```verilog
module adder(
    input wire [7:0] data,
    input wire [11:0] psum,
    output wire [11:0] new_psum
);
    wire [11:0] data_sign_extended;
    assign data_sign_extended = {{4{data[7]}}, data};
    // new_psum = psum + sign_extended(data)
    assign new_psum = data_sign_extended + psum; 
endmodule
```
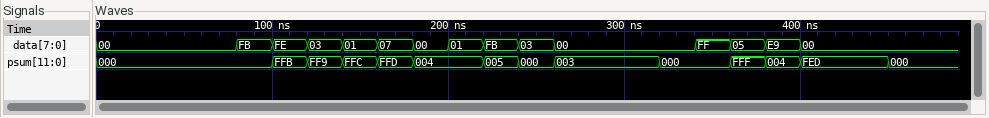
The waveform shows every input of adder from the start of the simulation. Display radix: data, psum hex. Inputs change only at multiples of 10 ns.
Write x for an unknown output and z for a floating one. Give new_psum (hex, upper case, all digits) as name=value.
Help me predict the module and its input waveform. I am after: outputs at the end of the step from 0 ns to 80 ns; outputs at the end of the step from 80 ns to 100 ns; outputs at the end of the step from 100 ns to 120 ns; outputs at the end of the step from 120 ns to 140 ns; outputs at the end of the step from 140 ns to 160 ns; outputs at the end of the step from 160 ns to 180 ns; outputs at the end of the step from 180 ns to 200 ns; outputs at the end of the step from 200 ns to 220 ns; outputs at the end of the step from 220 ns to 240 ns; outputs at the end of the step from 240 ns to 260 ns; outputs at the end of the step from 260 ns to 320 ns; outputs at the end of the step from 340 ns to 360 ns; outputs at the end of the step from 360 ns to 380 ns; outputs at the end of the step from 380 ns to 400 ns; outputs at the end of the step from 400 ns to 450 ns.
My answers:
new_psum=000
new_psum=FFB
new_psum=FF9
new_psum=FFC
new_psum=FFD
new_psum=004
new_psum=004
new_psum=005
new_psum=000
new_psum=003
new_psum=003
new_psum=FFF
new_psum=004
new_psum=FED
new_psum=FED
